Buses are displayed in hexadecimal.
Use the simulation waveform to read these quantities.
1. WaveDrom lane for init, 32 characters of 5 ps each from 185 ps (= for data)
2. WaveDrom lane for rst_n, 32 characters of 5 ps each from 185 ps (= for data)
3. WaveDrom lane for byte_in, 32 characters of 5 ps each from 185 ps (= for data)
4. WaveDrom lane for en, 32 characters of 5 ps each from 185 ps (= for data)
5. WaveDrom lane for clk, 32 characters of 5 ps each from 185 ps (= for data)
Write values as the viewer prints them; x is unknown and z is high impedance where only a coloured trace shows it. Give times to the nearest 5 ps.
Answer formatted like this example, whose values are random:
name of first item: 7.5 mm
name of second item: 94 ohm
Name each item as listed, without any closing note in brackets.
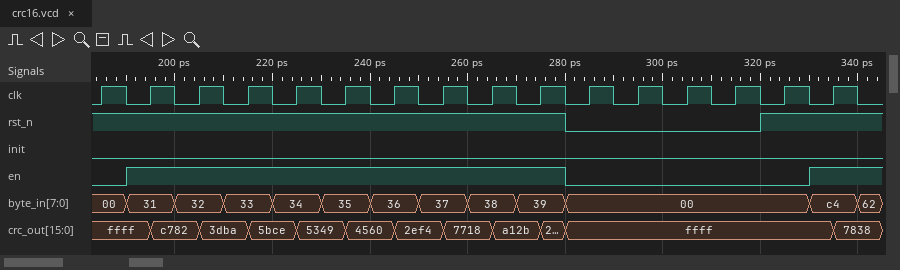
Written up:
WaveDrom lane for init, 32 characters of 5 ps each from 185 ps: {name: 'init', wave: '0...............................'}
WaveDrom lane for rst_n, 32 characters of 5 ps each from 185 ps: {name: 'rst_n', wave: '1..................0.......1....'}
WaveDrom lane for byte_in, 32 characters of 5 ps each from 185 ps: {name: 'byte_in', wave: '==.=.=.=.=.=.=.=.=.=.........=.=', data: '00 31 32 33 34 35 36 37 38 39 00 c4 62'}
WaveDrom lane for en, 32 characters of 5 ps each from 185 ps: {name: 'en', wave: '01.................0.........1..'}
WaveDrom lane for clk, 32 characters of 5 ps each from 185 ps: {name: 'clk', wave: '10101010101010101010101010101010'}
